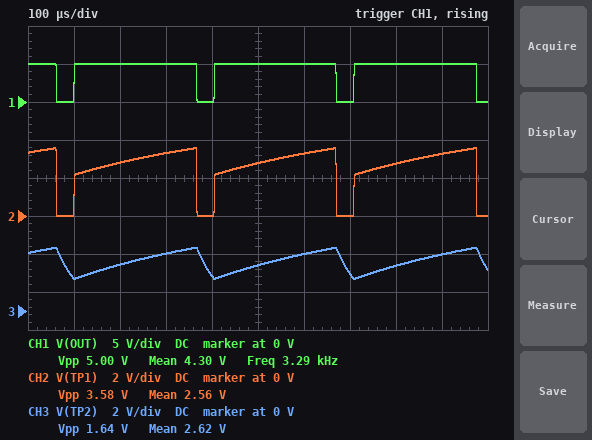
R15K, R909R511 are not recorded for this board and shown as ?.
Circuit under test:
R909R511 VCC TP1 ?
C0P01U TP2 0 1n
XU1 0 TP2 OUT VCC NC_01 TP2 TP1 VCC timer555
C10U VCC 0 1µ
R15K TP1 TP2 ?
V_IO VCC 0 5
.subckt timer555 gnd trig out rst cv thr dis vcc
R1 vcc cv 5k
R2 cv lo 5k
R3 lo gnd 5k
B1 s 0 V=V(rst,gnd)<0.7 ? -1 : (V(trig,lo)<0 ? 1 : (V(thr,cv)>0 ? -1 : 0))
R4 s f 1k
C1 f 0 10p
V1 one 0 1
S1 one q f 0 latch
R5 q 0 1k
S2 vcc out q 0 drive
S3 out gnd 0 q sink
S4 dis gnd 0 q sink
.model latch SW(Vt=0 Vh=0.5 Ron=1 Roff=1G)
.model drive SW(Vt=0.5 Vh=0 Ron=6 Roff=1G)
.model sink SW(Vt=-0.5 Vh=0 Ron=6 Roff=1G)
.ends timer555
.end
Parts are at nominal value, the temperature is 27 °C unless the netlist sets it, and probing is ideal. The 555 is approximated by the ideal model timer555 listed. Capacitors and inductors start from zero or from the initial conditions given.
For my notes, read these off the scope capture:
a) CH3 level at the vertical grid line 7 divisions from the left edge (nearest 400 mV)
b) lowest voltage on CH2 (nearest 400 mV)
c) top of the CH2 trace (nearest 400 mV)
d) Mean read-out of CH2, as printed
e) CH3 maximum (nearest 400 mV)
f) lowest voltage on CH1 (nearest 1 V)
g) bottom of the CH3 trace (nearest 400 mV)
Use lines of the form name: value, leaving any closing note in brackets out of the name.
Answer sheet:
CH3 level at the vertical grid line 7 divisions from the left edge: 2.0 V
lowest voltage on CH2: 0 V
top of the CH2 trace: 3.6 V
Mean read-out of CH2, as printed: 2.56 V
CH3 maximum: 3.2 V
lowest voltage on CH1: 0 V
bottom of the CH3 trace: 1.6 V
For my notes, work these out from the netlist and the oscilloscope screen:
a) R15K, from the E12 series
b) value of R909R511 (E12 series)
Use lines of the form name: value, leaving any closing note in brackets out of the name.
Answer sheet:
R15K, from the E12 series: 56 kΩ
value of R909R511: 330 kΩ
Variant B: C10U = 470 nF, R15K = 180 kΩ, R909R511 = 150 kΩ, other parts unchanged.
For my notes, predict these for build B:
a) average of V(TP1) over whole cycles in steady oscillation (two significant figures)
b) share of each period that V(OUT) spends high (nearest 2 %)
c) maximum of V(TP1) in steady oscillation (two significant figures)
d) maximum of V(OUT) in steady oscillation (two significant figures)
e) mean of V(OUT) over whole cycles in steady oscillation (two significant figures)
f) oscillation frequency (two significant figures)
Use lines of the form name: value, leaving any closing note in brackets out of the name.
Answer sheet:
average of V(TP1) over whole cycles in steady oscillation: 2.5 V
share of each period that V(OUT) spends high: 64 %
maximum of V(TP1) in steady oscillation: 4.2 V
maximum of V(OUT) in steady oscillation: 5.0 V
mean of V(OUT) over whole cycles in steady oscillation: 3.2 V
oscillation frequency: 2.8 kHz
